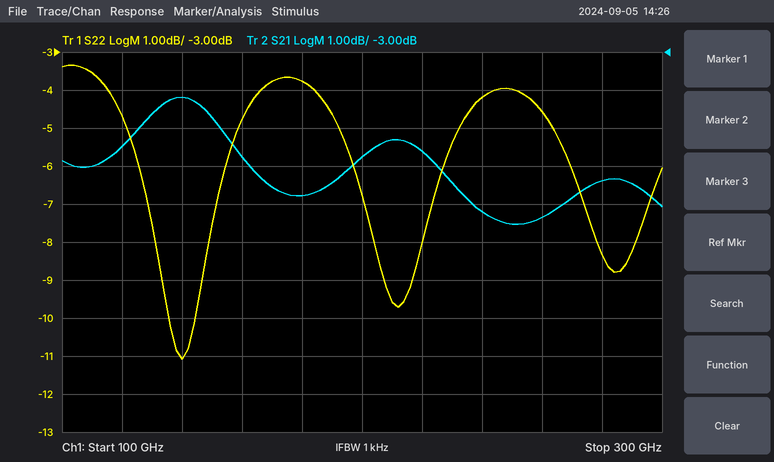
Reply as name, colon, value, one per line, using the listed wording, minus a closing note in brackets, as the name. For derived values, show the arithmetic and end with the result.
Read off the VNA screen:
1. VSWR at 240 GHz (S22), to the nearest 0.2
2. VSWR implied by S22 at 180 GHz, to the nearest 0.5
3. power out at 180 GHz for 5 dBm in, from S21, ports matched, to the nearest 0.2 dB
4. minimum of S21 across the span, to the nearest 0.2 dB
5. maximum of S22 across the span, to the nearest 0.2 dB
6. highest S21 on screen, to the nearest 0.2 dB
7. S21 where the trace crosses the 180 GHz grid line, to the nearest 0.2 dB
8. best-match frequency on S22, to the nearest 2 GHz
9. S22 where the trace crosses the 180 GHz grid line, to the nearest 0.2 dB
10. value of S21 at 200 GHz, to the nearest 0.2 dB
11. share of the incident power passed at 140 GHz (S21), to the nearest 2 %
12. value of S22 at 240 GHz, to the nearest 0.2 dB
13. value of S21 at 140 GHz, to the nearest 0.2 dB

VSWR at 240 GHz (S22), to the nearest 0.2: |Γ| = 10^(-4.2/20) = 0.6166; VSWR = (1 + 0.6166)/(1 − 0.6166) ≈ 4.2
VSWR implied by S22 at 180 GHz, to the nearest 0.5: |Γ| = 10^(-3.8/20) = 0.6457; VSWR = (1 + 0.6457)/(1 − 0.6457) ≈ 4.64, so 4.5 to the nearest 0.5
power out at 180 GHz for 5 dBm in, from S21, ports matched, to the nearest 0.2 dB: 5 dBm + (-6.8 dB) = -1.8 dBm
minimum of S21 across the span, to the nearest 0.2 dB: -7.6 dB
maximum of S22 across the span, to the nearest 0.2 dB: -3.4 dB
highest S21 on screen, to the nearest 0.2 dB: -4.2 dB
S21 where the trace crosses the 180 GHz grid line, to the nearest 0.2 dB: -6.8 dB
best-match frequency on S22, to the nearest 2 GHz: 140 GHz
S22 where the trace crosses the 180 GHz grid line, to the nearest 0.2 dB: -3.8 dB
value of S21 at 200 GHz, to the nearest 0.2 dB: -5.8 dB
share of the incident power passed at 140 GHz (S21), to the nearest 2 %: 10^(-4.2/10) ≈ 38 %
value of S22 at 240 GHz, to the nearest 0.2 dB: -4.2 dB
value of S21 at 140 GHz, to the nearest 0.2 dB: -4.2 dB
